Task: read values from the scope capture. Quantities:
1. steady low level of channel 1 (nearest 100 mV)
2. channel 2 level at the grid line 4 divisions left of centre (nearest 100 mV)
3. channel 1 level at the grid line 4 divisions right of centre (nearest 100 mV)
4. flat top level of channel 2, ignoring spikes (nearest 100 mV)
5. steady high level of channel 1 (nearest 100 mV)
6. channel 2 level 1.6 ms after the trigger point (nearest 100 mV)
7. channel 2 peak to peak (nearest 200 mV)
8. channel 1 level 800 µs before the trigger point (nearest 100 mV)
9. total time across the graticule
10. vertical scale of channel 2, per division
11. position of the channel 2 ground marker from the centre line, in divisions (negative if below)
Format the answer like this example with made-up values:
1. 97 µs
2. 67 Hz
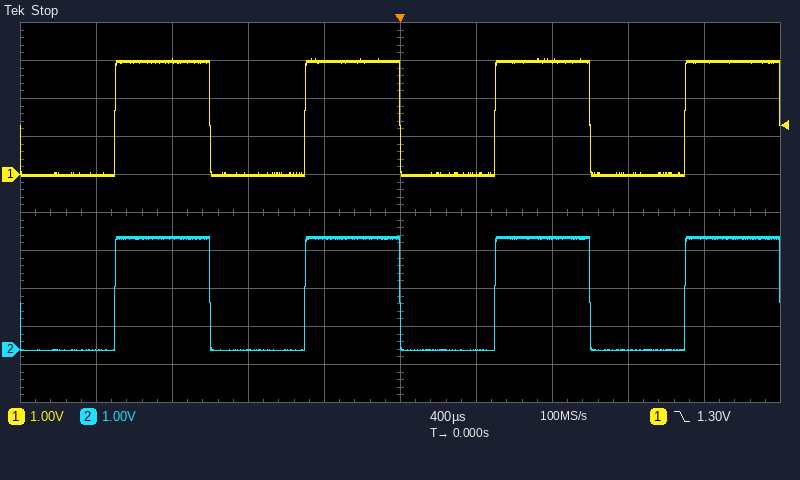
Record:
1. 0.0 V
2. 0.0 V
3. 3.0 V
4. 2.9 V
5. 3.0 V
6. 2.9 V
7. 3.0 V
8. 0.0 V
9. 4 ms
10. 1 V
11. -3.6 div
